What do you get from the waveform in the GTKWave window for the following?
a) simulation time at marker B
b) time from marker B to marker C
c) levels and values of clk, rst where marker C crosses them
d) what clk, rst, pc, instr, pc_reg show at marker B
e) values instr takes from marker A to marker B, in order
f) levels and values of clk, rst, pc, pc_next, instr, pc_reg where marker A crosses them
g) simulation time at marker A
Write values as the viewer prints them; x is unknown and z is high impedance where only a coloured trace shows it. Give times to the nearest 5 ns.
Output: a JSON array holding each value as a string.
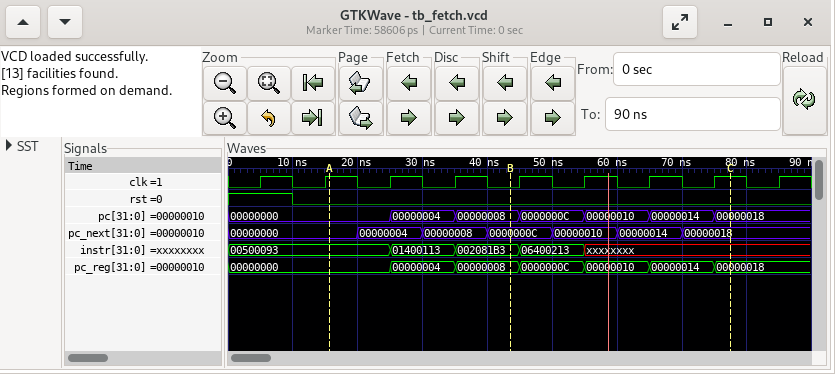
["45 ns", "35 ns", "clk=1, rst=0", "clk=0, rst=0, pc=00000008, instr=002081B3, pc_reg=00000008", "00500093, 01400113, 002081B3", "clk=1, rst=0, pc=00000000, pc_next=00000000, instr=00500093, pc_reg=00000000", "15 ns"]
